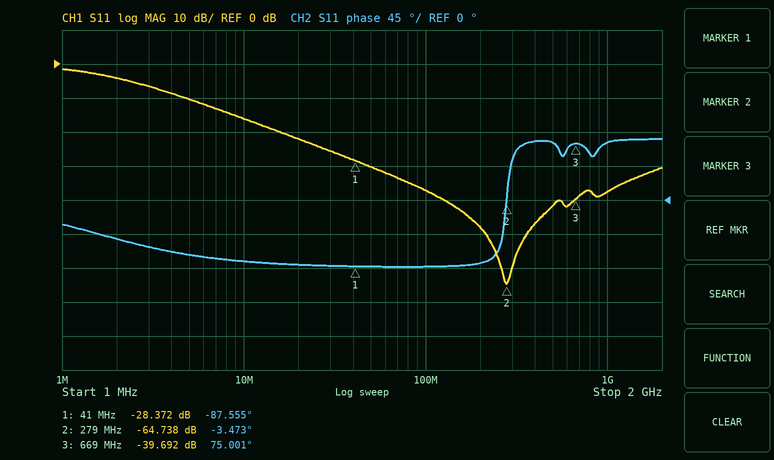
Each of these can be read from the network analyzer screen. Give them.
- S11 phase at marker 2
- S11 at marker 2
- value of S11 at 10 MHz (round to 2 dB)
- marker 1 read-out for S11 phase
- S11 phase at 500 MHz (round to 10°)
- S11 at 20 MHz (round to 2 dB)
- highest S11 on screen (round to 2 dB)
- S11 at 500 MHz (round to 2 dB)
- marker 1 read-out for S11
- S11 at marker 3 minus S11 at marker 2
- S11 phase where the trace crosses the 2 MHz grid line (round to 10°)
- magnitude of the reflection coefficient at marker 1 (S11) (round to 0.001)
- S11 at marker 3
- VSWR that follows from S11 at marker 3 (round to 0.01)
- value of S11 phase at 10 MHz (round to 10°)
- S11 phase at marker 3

-3.473°
-64.738 dB
-16 dB
-87.555°
80°
-22 dB
-2 dB
-42 dB
-28.372 dB
25.046 dB
-50°
0.038
-39.692 dB
1.02
-80°
75.001°
